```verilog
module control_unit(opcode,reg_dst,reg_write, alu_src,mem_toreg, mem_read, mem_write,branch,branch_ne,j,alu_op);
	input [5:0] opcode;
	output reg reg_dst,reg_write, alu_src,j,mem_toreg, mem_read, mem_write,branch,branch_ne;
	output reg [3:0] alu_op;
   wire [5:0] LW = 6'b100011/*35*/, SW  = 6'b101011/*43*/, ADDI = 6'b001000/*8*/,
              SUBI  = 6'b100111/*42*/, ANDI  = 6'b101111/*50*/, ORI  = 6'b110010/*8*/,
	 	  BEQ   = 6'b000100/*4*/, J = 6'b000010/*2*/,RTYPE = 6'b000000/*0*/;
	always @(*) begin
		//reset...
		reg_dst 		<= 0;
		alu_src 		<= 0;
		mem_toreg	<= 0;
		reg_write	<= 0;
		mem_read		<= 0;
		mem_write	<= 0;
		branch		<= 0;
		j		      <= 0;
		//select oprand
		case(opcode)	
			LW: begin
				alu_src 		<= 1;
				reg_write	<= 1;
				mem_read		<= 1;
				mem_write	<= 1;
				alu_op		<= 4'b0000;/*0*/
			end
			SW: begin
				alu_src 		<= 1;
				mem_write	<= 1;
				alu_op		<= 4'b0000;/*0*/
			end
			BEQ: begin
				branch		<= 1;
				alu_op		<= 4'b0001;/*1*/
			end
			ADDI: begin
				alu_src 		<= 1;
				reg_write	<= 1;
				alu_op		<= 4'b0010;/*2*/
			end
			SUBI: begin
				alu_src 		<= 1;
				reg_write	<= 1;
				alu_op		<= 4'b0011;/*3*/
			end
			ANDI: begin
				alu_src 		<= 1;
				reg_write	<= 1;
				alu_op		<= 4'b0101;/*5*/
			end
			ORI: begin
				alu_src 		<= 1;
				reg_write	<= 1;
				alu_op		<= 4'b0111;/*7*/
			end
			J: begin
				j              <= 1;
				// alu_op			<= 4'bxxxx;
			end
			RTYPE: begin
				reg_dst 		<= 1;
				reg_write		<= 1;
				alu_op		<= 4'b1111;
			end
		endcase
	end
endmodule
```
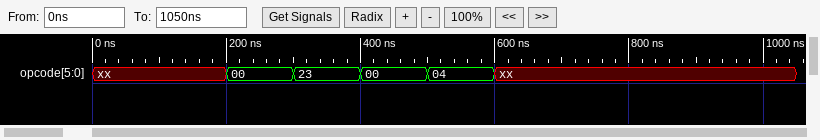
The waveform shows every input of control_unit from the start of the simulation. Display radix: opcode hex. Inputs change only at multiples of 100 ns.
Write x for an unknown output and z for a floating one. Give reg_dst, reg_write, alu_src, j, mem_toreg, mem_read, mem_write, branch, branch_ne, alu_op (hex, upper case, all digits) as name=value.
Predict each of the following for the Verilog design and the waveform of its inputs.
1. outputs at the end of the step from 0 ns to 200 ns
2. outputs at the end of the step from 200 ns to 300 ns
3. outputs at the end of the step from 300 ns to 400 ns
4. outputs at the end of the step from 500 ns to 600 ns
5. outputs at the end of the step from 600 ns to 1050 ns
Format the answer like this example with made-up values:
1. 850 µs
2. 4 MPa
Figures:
1. reg_dst=0, reg_write=0, alu_src=0, j=0, mem_toreg=0, mem_read=0, mem_write=0, branch=0, branch_ne=x, alu_op=x
2. reg_dst=1, reg_write=1, alu_src=0, j=0, mem_toreg=0, mem_read=0, mem_write=0, branch=0, branch_ne=x, alu_op=F
3. reg_dst=0, reg_write=1, alu_src=1, j=0, mem_toreg=0, mem_read=1, mem_write=1, branch=0, branch_ne=x, alu_op=0
4. reg_dst=0, reg_write=0, alu_src=0, j=0, mem_toreg=0, mem_read=0, mem_write=0, branch=1, branch_ne=x, alu_op=1
5. reg_dst=0, reg_write=0, alu_src=0, j=0, mem_toreg=0, mem_read=0, mem_write=0, branch=0, branch_ne=x, alu_op=1
